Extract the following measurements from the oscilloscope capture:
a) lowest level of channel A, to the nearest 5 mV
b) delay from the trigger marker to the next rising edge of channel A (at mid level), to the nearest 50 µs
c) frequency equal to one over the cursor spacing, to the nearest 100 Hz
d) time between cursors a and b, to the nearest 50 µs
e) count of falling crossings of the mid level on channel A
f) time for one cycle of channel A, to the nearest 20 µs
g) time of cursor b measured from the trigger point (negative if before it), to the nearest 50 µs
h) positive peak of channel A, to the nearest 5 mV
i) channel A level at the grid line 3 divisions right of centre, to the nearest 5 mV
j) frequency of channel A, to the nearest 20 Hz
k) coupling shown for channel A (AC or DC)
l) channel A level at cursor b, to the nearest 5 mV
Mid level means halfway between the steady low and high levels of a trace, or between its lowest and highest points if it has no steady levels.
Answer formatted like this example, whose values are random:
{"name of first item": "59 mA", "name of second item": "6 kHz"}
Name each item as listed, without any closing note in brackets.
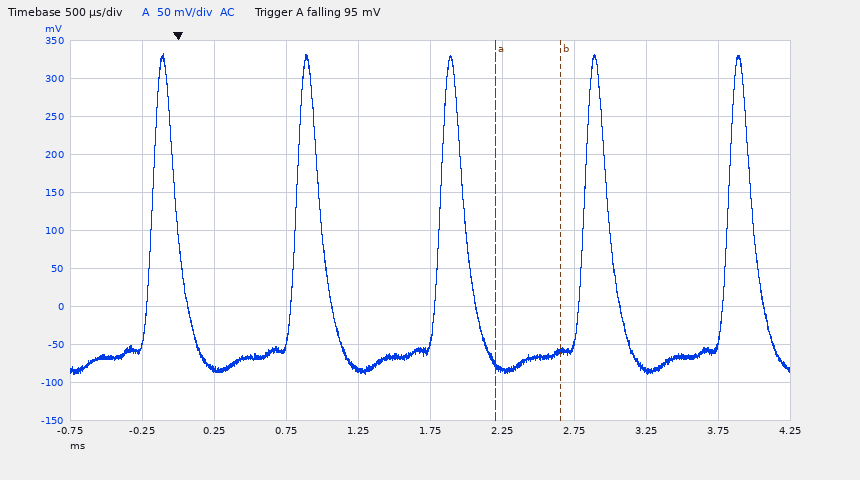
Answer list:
{"lowest level of channel A, to the nearest 5 mV": "-90 mV", "delay from the trigger marker to the next rising edge of channel A (at mid level), to the nearest 50 µs": "800 µs", "frequency equal to one over the cursor spacing, to the nearest 100 Hz": "2.2 kHz", "time between cursors a and b, to the nearest 50 µs": "450 µs", "count of falling crossings of the mid level on channel A": "5", "time for one cycle of channel A, to the nearest 20 µs": "1.00 ms", "time of cursor b measured from the trigger point (negative if before it), to the nearest 50 µs": "+2.65 ms", "positive peak of channel A, to the nearest 5 mV": "335 mV", "channel A level at the grid line 3 divisions right of centre, to the nearest 5 mV": "-85 mV", "frequency of channel A, to the nearest 20 Hz": "1.00 kHz", "coupling shown for channel A": "AC", "channel A level at cursor b, to the nearest 5 mV": "-60 mV"}
